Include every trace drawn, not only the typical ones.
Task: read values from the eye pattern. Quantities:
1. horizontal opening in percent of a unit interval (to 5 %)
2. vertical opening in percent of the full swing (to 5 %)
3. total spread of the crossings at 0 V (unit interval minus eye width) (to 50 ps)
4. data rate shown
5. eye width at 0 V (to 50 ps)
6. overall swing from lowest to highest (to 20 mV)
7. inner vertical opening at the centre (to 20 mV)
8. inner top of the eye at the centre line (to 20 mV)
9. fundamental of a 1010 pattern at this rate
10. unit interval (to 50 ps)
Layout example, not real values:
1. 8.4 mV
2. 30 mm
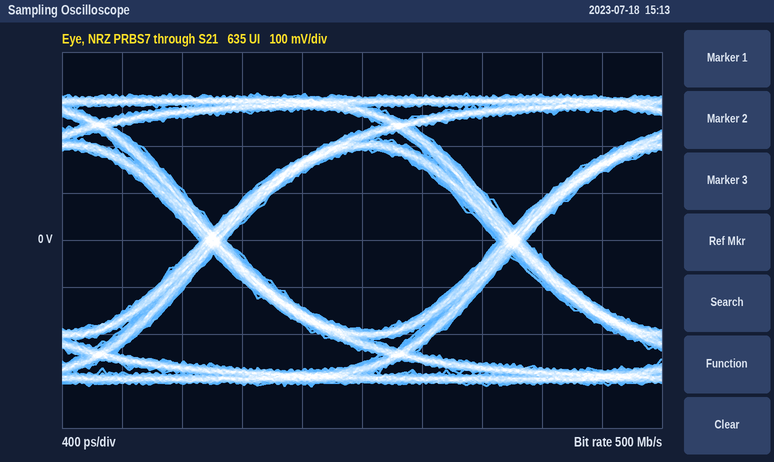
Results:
1. 90 %
2. 60 %
3. 200 ps
4. 500 Mb/s
5. 1.80 ns
6. 620 mV
7. 380 mV
8. 200 mV
9. 250 MHz
10. 2.00 ns
